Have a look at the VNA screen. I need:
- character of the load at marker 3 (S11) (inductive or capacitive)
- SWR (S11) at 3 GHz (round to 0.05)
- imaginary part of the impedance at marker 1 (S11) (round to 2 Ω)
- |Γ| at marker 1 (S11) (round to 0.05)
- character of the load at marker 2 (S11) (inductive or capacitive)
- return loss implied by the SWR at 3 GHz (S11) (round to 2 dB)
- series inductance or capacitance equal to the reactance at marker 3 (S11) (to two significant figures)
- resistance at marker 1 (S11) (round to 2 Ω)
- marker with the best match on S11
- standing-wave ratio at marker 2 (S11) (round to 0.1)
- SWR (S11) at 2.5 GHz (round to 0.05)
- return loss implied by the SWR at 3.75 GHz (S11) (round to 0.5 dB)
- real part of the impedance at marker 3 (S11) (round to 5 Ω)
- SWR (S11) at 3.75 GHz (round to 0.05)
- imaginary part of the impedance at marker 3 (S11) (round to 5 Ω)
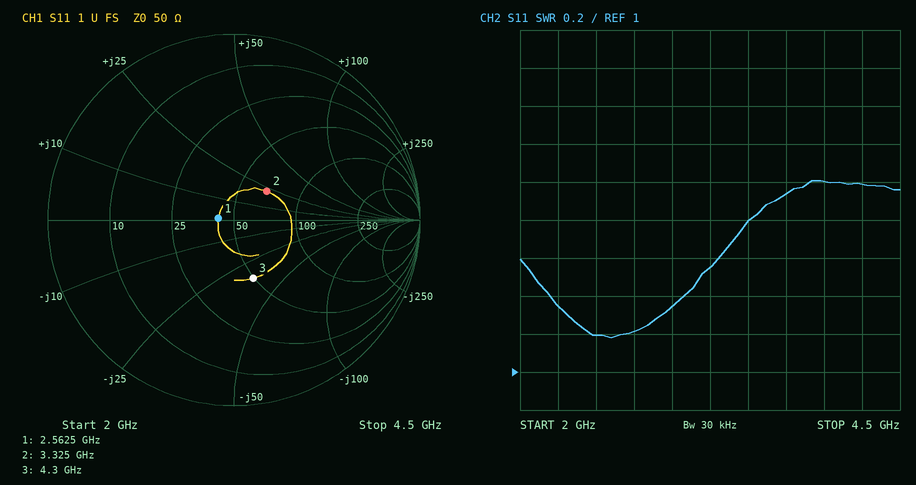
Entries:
capacitive
1.35
0 Ω
0.10
inductive
16 dB
1.1 pF
42 Ω
marker 1
1.6
1.20
10.0 dB
50 Ω
1.95
-35 Ω
